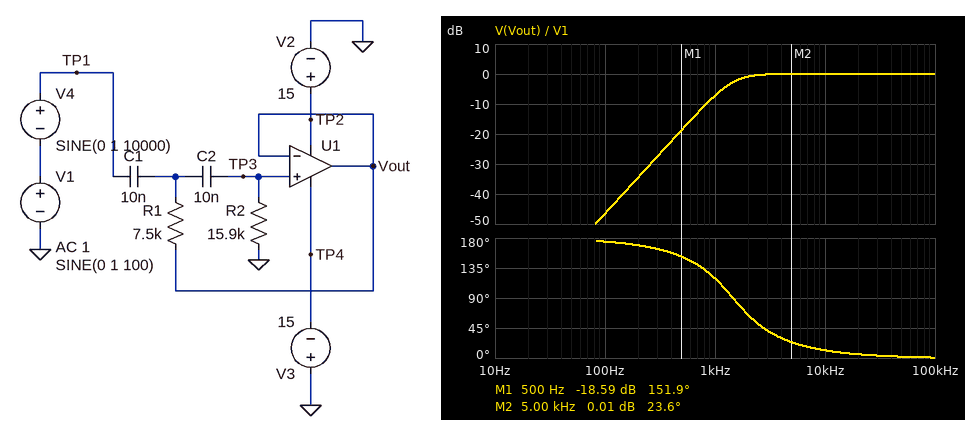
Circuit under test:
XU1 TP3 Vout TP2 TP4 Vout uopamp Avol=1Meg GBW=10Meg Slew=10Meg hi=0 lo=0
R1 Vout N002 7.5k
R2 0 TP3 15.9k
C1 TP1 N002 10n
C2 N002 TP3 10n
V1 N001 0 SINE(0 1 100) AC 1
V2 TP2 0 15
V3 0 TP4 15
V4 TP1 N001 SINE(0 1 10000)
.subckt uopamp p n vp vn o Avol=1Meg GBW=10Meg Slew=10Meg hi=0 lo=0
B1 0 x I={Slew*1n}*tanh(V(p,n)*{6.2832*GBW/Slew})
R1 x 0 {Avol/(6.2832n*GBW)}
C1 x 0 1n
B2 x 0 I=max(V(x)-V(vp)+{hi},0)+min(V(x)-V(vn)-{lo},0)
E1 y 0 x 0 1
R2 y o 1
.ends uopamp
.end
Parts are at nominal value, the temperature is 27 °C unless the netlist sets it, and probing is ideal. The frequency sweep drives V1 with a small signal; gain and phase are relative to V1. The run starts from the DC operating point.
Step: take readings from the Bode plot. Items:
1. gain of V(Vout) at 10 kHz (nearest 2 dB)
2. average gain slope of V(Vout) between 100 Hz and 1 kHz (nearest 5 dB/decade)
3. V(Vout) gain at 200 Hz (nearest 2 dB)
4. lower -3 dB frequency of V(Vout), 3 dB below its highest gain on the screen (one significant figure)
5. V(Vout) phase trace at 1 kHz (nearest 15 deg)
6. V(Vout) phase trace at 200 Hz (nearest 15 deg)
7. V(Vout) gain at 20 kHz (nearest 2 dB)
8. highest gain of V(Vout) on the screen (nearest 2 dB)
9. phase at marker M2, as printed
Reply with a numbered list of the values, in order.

1. 0 dB
2. 40 dB/decade
3. -34 dB
4. 1 kHz
5. 120 deg
6. 165 deg
7. 0 dB
8. 0 dB
9. 23.6 deg
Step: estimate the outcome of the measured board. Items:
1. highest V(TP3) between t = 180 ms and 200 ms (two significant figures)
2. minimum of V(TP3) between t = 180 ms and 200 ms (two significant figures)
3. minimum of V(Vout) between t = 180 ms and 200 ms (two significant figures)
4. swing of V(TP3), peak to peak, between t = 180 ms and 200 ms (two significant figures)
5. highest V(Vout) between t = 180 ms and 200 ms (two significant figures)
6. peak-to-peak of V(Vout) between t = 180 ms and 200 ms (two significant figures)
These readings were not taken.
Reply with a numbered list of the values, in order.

1. 1.0 V
2. -1.0 V
3. -1.0 V
4. 2.0 V
5. 1.0 V
6. 2.0 V
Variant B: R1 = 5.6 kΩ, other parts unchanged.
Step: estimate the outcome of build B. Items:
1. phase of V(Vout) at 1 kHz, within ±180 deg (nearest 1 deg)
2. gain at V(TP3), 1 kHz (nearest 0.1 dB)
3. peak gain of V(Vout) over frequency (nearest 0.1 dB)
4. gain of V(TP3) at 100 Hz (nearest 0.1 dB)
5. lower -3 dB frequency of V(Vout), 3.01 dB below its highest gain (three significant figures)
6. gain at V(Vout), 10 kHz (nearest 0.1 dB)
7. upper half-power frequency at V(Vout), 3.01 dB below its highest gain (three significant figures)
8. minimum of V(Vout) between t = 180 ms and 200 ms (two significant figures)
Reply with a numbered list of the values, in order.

1. 133 deg
2. -8.7 dB
3. 0.4 dB
4. -49.1 dB
5. 1.51 kHz
6. 0.1 dB
7. 9.08 MHz
8. -1.0 V
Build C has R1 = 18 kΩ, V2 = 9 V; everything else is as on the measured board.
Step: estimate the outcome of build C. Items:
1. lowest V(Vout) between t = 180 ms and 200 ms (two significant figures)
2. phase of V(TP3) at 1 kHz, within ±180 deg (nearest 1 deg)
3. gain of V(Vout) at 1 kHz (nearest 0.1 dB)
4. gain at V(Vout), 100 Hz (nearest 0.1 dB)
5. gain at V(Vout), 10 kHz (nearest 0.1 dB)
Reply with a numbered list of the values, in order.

1. -1.0 V
2. 87 deg
3. -6.0 dB
4. -39.1 dB
5. -0.1 dB
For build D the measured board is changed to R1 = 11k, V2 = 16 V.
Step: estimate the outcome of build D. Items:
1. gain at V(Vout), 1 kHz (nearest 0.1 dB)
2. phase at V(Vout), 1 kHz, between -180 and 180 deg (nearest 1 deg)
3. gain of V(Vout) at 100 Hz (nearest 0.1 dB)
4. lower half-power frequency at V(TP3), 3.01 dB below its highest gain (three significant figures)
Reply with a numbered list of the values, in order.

1. -6.2 dB
2. 103 deg
3. -43.2 dB
4. 1.45 kHz
